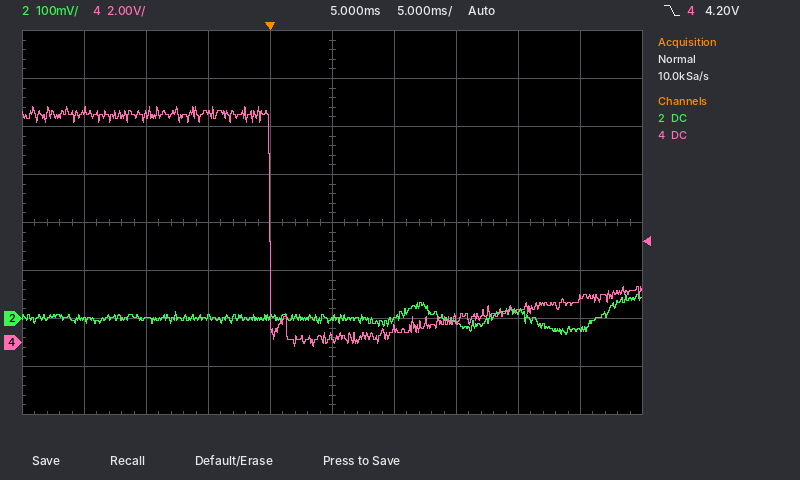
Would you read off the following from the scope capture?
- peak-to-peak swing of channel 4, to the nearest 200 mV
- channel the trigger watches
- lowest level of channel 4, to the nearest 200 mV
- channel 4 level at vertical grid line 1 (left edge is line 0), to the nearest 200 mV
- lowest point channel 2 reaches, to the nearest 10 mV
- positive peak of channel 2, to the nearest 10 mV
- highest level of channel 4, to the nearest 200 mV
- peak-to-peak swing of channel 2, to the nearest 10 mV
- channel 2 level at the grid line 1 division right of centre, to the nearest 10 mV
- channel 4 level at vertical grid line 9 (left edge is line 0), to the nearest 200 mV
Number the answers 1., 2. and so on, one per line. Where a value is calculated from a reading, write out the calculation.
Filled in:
1. 9.8 V − (-200 mV) = 10.0 V
2. channel 4
3. -200 mV
4. 9.6 V
5. -30 mV
6. 50 mV
7. 9.8 V
8. 50 mV − (-30 mV) = 80 mV
9. 0 mV
10. 1.8 V
